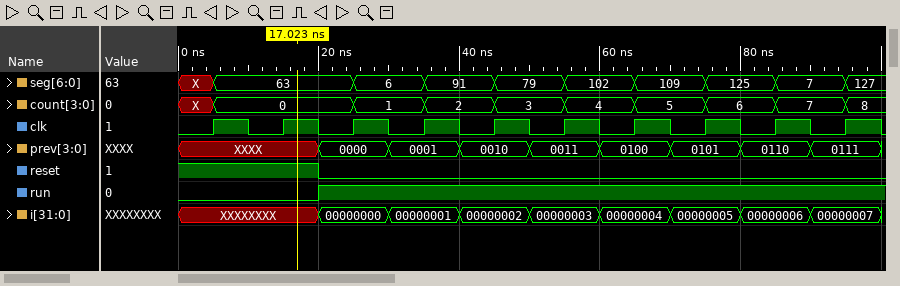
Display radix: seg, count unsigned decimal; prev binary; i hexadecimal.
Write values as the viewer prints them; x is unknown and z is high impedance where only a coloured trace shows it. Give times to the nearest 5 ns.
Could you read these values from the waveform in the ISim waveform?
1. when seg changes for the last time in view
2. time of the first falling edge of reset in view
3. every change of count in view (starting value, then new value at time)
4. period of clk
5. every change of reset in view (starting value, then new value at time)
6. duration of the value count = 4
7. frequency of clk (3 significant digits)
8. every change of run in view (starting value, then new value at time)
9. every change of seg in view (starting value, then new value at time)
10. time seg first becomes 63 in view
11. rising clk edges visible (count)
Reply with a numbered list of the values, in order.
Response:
1. 95 ns
2. 20 ns
3. X, 0 at 5 ns, 1 at 25 ns, 2 at 35 ns, 3 at 45 ns, 4 at 55 ns, 5 at 65 ns, 6 at 75 ns, 7 at 85 ns, 8 at 95 ns
4. 10 ns
5. 1, 0 at 20 ns
6. 10 ns
7. 100 MHz
8. 0, 1 at 20 ns
9. X, 63 at 5 ns, 6 at 25 ns, 91 at 35 ns, 79 at 45 ns, 102 at 55 ns, 109 at 65 ns, 125 at 75 ns, 7 at 85 ns, 127 at 95 ns
10. 5 ns
11. 10
